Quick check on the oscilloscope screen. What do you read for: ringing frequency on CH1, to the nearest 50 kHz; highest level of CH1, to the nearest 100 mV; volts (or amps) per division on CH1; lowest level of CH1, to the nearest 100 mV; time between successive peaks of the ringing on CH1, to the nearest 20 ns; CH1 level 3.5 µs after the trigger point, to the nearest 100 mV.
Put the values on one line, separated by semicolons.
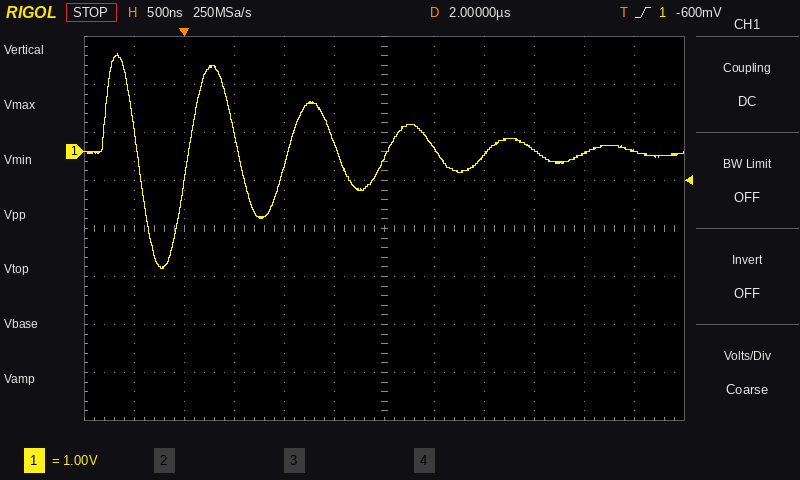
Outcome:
1.00 MHz; 2.0 V; 1 V; -2.4 V; 980 ns; 0.0 V
